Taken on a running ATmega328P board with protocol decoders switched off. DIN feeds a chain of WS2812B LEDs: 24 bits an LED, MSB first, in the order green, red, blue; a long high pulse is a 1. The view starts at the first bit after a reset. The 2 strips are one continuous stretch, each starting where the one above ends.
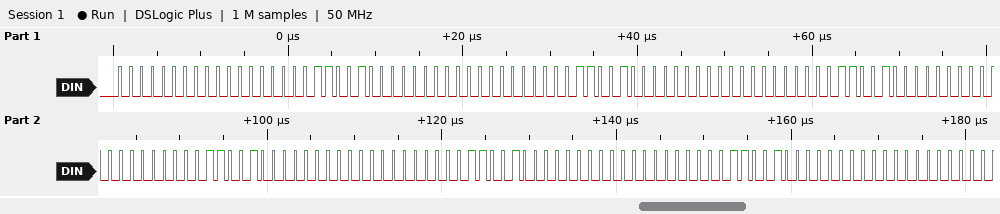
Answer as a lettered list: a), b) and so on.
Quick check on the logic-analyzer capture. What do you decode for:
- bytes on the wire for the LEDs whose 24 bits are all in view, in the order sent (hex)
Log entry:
a) 00 00 32 00 00 32 00 00 32 00 00 32 00 00 32 00 00 32
